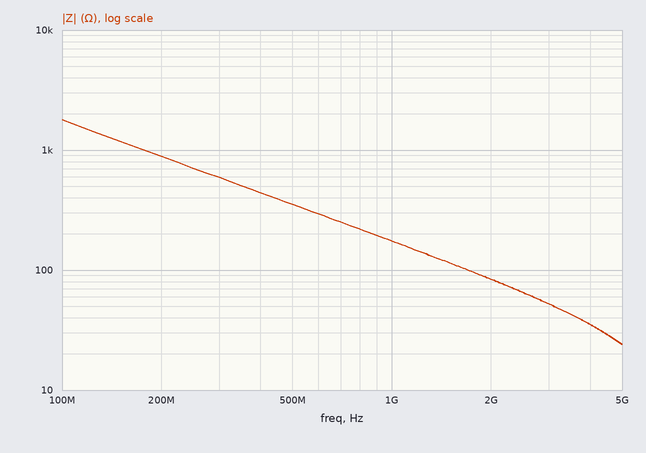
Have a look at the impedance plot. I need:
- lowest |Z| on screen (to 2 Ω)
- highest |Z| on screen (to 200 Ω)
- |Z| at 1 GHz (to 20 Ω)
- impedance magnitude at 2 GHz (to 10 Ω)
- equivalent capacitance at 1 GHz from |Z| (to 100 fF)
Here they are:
24 Ω
1.8 kΩ
180 Ω
80 Ω
900 fF
